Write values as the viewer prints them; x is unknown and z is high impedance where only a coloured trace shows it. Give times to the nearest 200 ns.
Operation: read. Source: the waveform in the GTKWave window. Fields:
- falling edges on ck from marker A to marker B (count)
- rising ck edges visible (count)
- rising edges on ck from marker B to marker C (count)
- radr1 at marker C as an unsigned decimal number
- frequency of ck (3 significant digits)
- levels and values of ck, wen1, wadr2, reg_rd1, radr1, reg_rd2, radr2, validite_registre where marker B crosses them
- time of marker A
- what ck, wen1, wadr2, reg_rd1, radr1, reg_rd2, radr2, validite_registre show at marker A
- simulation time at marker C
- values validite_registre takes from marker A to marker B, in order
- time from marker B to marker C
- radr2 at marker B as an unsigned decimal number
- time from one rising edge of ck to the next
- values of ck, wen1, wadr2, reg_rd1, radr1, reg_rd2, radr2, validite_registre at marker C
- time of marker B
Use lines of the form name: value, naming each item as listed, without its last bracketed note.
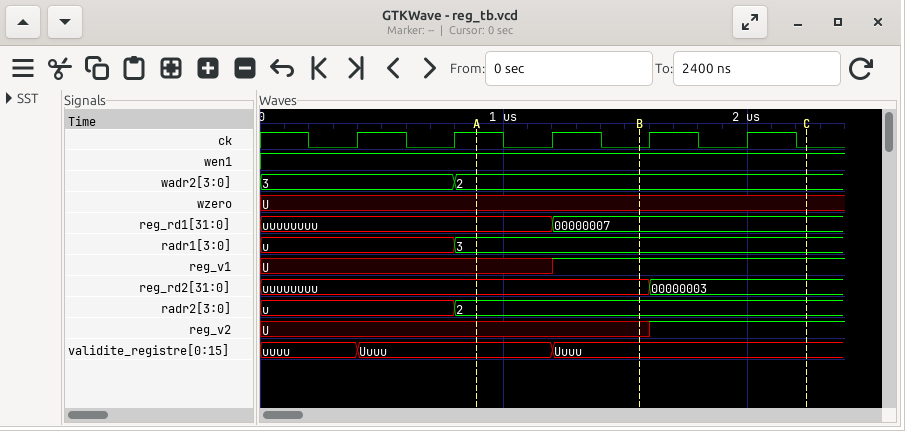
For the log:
falling edges on ck from marker A to marker B: 2
rising ck edges visible: 5
rising edges on ck from marker B to marker C: 2
radr1 at marker C as an unsigned decimal number: 3
frequency of ck: 2.50 MHz
levels and values of ck, wen1, wadr2, reg_rd1, radr1, reg_rd2, radr2, validite_registre where marker B crosses them: ck=0, wen1=1, wadr2=2, reg_rd1=00000007, radr1=3, reg_rd2=uuuuuuuu, radr2=2, validite_registre=Uuuu
time of marker A: 800 ns
what ck, wen1, wadr2, reg_rd1, radr1, reg_rd2, radr2, validite_registre show at marker A: ck=1, wen1=1, wadr2=2, reg_rd1=uuuuuuuu, radr1=3, reg_rd2=uuuuuuuu, radr2=2, validite_registre=Uuuu
simulation time at marker C: 2200 ns
values validite_registre takes from marker A to marker B, in order: Uuuu, Uuuu
time from marker B to marker C: 600 ns
radr2 at marker B as an unsigned decimal number: 2
time from one rising edge of ck to the next: 400 ns
values of ck, wen1, wadr2, reg_rd1, radr1, reg_rd2, radr2, validite_registre at marker C: ck=0, wen1=1, wadr2=2, reg_rd1=00000007, radr1=3, reg_rd2=00000003, radr2=2, validite_registre=Uuuu
time of marker B: 1600 ns
